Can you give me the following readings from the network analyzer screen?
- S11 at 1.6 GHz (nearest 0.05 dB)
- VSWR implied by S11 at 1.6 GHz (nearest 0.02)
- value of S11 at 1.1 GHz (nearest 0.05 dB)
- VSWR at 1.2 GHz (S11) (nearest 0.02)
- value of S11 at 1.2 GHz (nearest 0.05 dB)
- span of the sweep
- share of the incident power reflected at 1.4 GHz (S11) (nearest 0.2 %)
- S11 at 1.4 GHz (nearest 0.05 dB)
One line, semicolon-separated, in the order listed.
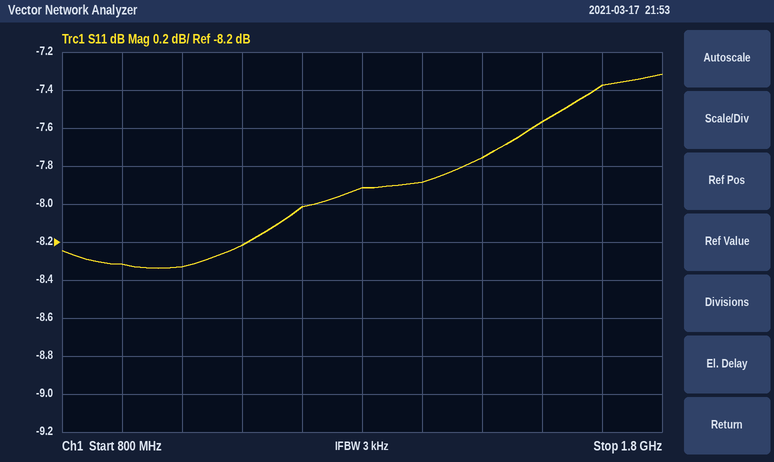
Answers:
-7.55 dB; 2.44; -8.20 dB; 2.32; -8.00 dB; 1 GHz; 16.2 %; -7.90 dB
